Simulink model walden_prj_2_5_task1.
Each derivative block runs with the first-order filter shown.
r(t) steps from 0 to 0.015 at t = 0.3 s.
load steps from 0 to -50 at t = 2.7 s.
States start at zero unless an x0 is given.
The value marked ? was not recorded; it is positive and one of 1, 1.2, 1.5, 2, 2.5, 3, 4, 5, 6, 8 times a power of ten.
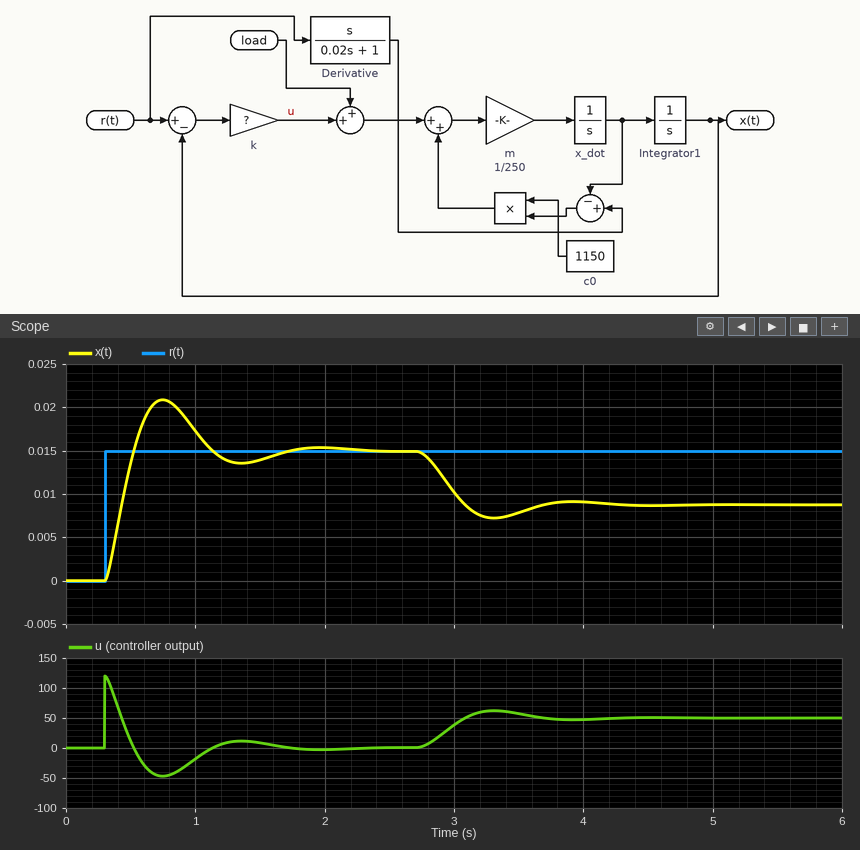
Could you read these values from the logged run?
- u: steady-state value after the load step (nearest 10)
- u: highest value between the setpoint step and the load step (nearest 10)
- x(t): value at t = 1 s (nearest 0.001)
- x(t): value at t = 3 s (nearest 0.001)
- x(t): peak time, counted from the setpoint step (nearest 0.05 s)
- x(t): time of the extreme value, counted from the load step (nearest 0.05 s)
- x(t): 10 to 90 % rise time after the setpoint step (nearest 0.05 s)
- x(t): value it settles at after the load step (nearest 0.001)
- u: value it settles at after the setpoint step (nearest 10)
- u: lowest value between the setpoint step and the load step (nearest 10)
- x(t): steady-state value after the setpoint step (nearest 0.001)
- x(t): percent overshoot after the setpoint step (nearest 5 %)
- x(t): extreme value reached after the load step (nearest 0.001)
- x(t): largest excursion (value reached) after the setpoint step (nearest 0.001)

50
120
0.017
0.010
0.45 s
0.60 s
0.15 s
0.009
0
-50
0.015
40 %
0.007
0.021
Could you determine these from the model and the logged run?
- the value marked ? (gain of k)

8000
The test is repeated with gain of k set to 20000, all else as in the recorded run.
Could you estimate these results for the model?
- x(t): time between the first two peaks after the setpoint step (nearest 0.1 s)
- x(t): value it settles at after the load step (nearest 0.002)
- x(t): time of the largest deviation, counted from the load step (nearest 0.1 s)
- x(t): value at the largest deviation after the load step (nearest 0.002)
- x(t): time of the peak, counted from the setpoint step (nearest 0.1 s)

0.7 s
0.012
0.4 s
0.012
0.3 s
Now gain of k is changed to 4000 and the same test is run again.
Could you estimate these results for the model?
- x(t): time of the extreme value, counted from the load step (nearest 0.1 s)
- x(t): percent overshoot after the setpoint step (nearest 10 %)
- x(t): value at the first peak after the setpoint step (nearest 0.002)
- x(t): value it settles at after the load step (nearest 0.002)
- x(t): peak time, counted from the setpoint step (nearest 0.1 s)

1.0 s
30 %
0.020
0.002
0.6 s
